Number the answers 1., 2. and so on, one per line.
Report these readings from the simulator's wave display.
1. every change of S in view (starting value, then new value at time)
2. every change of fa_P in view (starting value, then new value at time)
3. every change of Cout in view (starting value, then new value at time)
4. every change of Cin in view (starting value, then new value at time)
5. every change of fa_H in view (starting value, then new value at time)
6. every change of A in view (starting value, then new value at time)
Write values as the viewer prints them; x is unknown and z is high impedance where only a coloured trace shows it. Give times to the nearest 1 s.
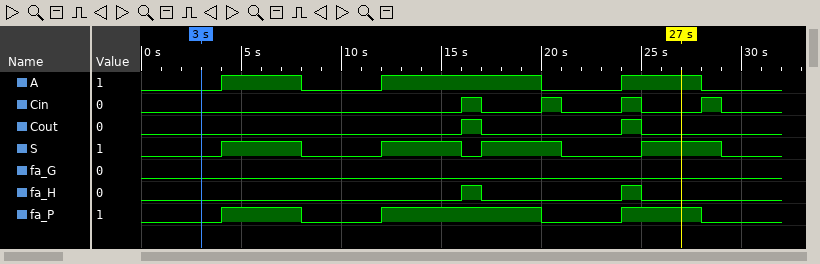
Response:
1. 0, 1 at 4 s, 0 at 8 s, 1 at 12 s, 0 at 16 s, 1 at 17 s, 0 at 21 s, 1 at 25 s, 0 at 29 s
2. 0, 1 at 4 s, 0 at 8 s, 1 at 12 s, 0 at 20 s, 1 at 24 s, 0 at 28 s
3. 0, 1 at 16 s, 0 at 17 s, 1 at 24 s, 0 at 25 s
4. 0, 1 at 16 s, 0 at 17 s, 1 at 20 s, 0 at 21 s, 1 at 24 s, 0 at 25 s, 1 at 28 s, 0 at 29 s
5. 0, 1 at 16 s, 0 at 17 s, 1 at 24 s, 0 at 25 s
6. 0, 1 at 4 s, 0 at 8 s, 1 at 12 s, 0 at 20 s, 1 at 24 s, 0 at 28 s
